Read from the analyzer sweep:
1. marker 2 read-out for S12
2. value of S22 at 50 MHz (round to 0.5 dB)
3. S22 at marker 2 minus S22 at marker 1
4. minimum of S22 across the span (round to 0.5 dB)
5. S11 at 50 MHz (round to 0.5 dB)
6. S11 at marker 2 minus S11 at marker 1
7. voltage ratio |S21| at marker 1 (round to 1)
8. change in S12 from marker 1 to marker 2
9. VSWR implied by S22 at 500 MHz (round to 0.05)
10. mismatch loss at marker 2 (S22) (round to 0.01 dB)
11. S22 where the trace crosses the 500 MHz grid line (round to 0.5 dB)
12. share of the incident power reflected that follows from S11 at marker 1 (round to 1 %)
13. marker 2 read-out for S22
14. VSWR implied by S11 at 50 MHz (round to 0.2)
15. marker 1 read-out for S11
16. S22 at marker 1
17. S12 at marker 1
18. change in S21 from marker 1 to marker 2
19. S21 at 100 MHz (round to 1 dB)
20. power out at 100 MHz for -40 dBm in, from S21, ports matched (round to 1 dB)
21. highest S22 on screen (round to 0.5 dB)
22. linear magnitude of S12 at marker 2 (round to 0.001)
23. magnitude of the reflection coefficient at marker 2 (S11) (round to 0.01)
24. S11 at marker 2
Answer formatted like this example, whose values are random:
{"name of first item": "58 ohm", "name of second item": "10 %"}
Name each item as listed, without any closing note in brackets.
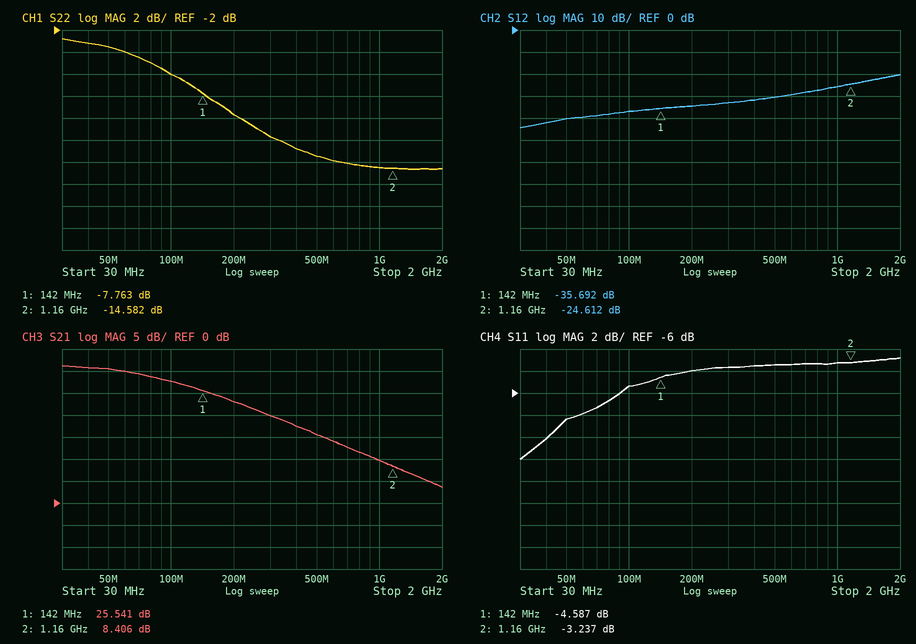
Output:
{"marker 2 read-out for S12": "-24.612 dB", "value of S22 at 50 MHz": "-3.5 dB", "S22 at marker 2 minus S22 at marker 1": "-6.819 dB", "minimum of S22 across the span": "-14.5 dB", "S11 at 50 MHz": "-8.5 dB", "S11 at marker 2 minus S11 at marker 1": "1.350 dB", "voltage ratio |S21| at marker 1": "19", "change in S12 from marker 1 to marker 2": "11.080 dB", "VSWR implied by S22 at 500 MHz": "1.55", "mismatch loss at marker 2 (S22)": "0.15 dB", "S22 where the trace crosses the 500 MHz grid line": "-13.5 dB", "share of the incident power reflected that follows from S11 at marker 1": "35 %", "marker 2 read-out for S22": "-14.582 dB", "VSWR implied by S11 at 50 MHz": "2.2", "marker 1 read-out for S11": "-4.587 dB", "S22 at marker 1": "-7.763 dB", "S12 at marker 1": "-35.692 dB", "change in S21 from marker 1 to marker 2": "-17.135 dB", "S21 at 100 MHz": "28 dB", "power out at 100 MHz for -40 dBm in, from S21, ports matched": "-12 dBm", "highest S22 on screen": "-3.0 dB", "linear magnitude of S12 at marker 2": "0.059", "magnitude of the reflection coefficient at marker 2 (S11)": "0.69", "S11 at marker 2": "-3.237 dB"}
